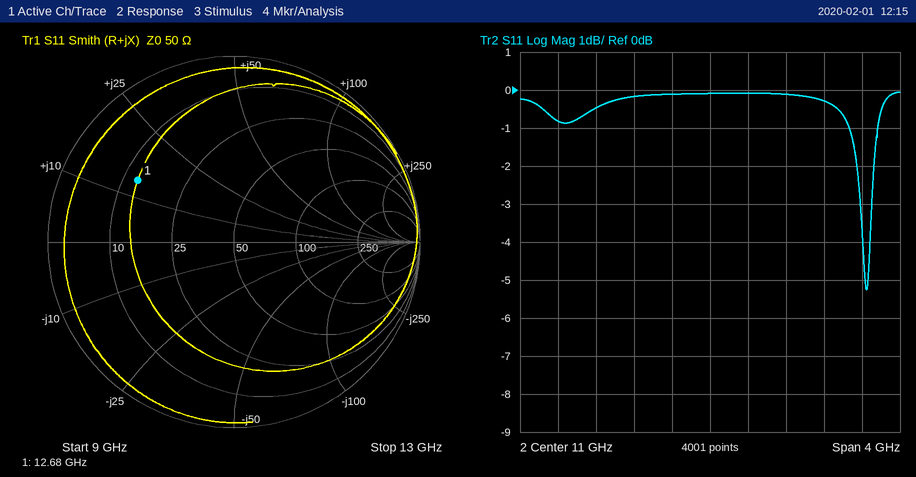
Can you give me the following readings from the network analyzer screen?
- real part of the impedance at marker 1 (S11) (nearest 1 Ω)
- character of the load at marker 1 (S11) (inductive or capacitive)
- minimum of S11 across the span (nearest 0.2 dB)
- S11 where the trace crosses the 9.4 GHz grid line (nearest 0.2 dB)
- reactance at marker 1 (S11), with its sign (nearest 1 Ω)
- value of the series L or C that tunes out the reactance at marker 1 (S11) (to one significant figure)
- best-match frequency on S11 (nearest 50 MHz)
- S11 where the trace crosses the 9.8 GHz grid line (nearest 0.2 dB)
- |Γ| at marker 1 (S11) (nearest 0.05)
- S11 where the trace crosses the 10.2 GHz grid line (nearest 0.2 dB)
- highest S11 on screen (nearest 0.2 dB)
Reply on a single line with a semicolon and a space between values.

13 Ω; inductive; -5.2 dB; -0.8 dB; +14 Ω; 900 fF; 12.65 GHz; -0.4 dB; 0.60; -0.2 dB; 0.0 dB
